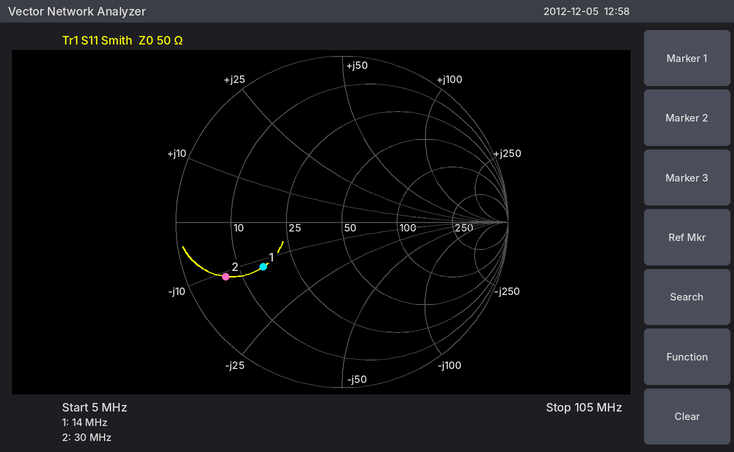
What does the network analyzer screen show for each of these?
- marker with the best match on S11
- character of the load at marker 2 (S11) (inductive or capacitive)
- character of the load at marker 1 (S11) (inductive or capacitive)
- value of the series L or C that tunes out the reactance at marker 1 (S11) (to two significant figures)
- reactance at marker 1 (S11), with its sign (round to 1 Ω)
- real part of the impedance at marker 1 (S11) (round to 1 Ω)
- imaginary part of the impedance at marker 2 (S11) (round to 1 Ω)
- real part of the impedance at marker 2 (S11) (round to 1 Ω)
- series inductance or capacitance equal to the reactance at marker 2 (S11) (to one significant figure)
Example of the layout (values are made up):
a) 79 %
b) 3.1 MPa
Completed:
a) marker 1
b) capacitive
c) capacitive
d) 140 nH
e) -12 Ω
f) 16 Ω
g) -11 Ω
h) 7 Ω
i) 500 pF
